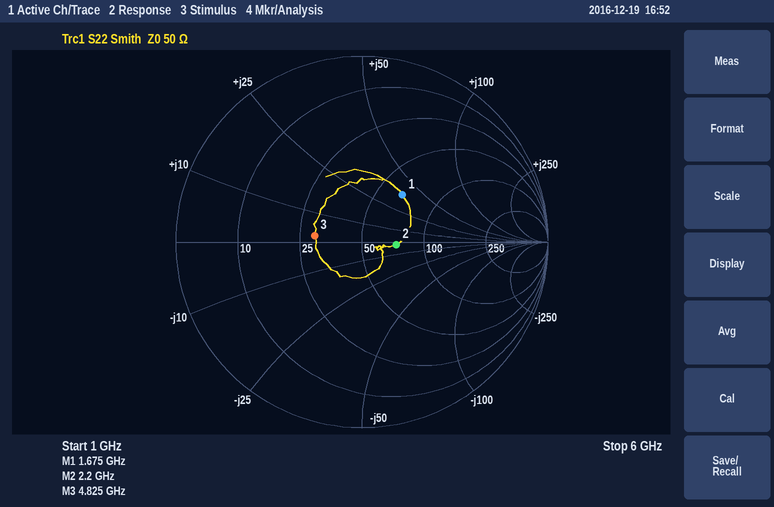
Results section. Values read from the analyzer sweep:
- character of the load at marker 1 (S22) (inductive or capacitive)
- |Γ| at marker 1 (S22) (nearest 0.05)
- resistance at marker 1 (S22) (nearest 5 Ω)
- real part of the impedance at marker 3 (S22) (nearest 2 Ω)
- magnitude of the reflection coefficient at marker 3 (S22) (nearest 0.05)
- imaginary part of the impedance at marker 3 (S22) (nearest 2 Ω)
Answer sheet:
inductive
0.35
65 Ω
30 Ω
0.25
+2 Ω
